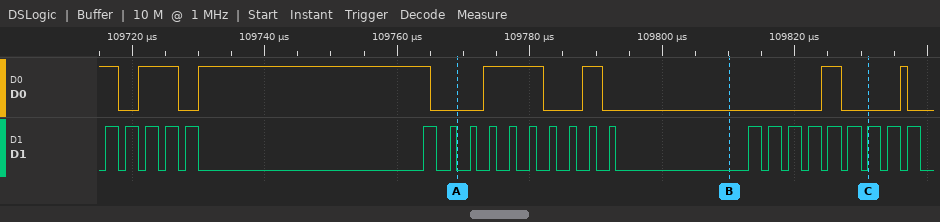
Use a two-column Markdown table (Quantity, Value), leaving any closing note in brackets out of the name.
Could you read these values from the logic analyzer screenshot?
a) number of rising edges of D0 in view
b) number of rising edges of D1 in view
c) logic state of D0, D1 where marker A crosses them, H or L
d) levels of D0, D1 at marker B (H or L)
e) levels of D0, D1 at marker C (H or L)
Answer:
| Quantity | Value |
|---|---|
| number of rising edges of D0 in view | 6 |
| number of rising edges of D1 in view | 24 |
| logic state of D0, D1 where marker A crosses them, H or L | D0=L, D1=L |
| levels of D0, D1 at marker B | D0=L, D1=L |
| levels of D0, D1 at marker C | D0=L, D1=H |
